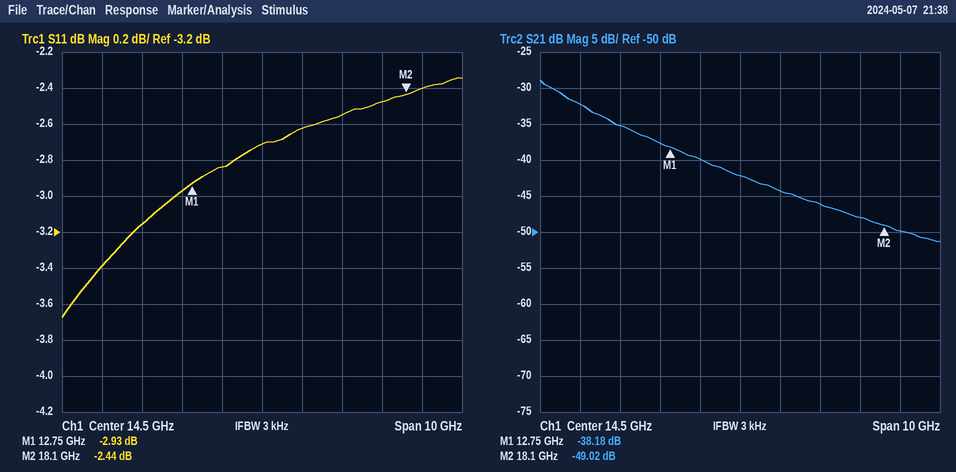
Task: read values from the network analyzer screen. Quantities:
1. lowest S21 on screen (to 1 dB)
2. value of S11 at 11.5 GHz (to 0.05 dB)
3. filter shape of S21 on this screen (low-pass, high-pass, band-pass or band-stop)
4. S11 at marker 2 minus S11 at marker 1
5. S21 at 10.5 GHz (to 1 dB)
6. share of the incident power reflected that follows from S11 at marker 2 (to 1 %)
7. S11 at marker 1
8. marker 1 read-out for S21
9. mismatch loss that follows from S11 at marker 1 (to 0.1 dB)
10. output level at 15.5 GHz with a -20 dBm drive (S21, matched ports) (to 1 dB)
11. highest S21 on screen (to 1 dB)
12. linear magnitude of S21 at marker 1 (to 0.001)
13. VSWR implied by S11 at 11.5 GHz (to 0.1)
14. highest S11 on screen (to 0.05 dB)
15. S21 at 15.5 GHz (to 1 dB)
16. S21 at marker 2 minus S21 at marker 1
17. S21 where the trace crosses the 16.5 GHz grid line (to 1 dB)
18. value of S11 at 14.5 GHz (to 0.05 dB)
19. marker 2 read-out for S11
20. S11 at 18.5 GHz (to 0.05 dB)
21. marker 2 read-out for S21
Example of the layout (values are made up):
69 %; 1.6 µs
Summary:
-51 dB; -3.15 dB; low-pass; 0.49 dB; -32 dB; 57 %; -2.93 dB; -38.18 dB; 3.1 dB; -64 dBm; -29 dB; 0.012; 5.6; -2.35 dB; -44 dB; -10.84 dB; -46 dB; -2.70 dB; -2.44 dB; -2.40 dB; -49.02 dB
